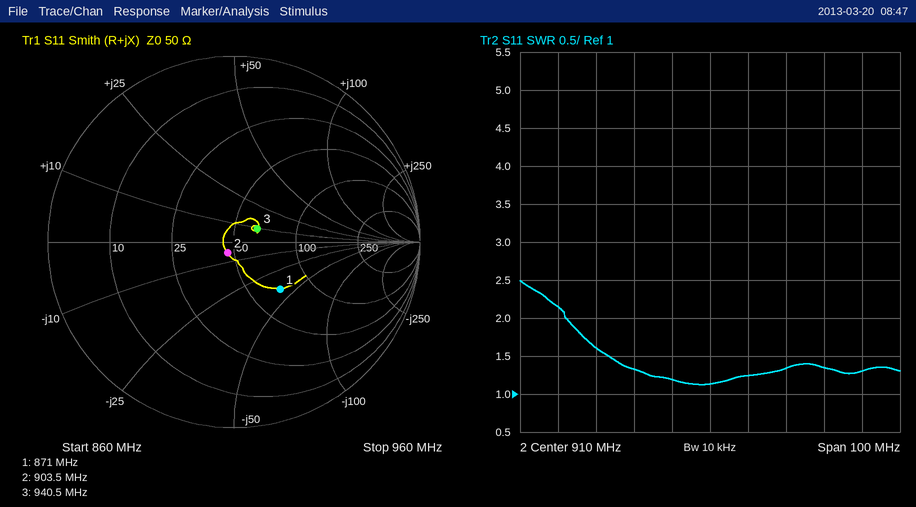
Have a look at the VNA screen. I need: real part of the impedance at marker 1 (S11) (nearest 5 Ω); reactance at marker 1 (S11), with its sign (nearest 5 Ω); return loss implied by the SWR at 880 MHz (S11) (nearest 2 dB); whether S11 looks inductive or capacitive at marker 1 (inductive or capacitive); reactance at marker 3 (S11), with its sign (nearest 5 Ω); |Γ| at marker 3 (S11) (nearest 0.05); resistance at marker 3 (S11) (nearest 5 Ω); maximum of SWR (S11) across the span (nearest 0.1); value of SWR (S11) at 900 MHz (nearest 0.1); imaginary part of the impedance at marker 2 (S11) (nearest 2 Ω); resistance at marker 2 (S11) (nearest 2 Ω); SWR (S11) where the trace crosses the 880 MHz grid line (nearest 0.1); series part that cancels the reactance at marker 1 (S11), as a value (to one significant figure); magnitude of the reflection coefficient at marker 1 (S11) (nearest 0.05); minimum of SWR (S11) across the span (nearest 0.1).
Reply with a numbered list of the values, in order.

1. 70 Ω
2. -40 Ω
3. 12 dB
4. capacitive
5. +10 Ω
6. 0.15
7. 65 Ω
8. 2.5
9. 1.2
10. -6 Ω
11. 46 Ω
12. 1.6
13. 7 nH
14. 0.35
15. 1.1
